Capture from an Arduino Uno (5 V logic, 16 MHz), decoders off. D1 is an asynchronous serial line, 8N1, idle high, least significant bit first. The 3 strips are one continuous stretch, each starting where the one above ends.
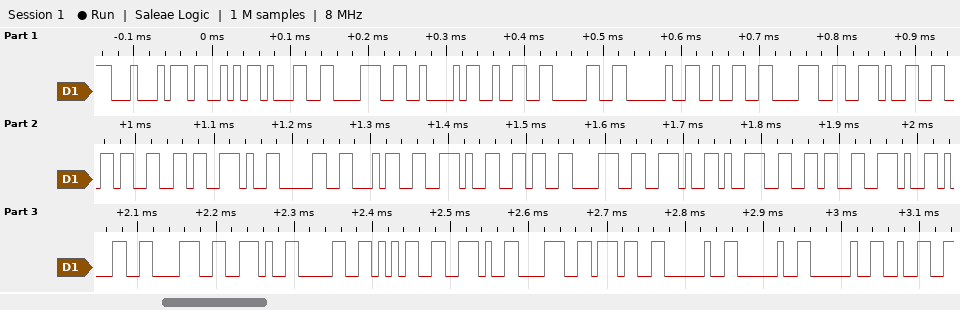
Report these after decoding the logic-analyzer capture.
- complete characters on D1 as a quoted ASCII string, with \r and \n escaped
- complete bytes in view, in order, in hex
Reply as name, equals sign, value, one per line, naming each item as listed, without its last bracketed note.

complete characters on D1 as a quoted ASCII string, with \r and \n escaped = "DS18B20 28.ff.04.68.96.18.05.87   2"
complete bytes in view, in order, in hex = 44 53 31 38 42 32 30 20 32 38 2E 66 66 2E 30 34 2E 36 38 2E 39 36 2E 31 38 2E 30 35 2E 38 37 20 20 20 32
